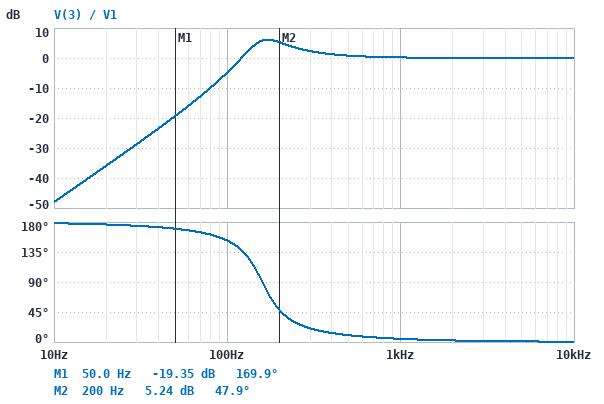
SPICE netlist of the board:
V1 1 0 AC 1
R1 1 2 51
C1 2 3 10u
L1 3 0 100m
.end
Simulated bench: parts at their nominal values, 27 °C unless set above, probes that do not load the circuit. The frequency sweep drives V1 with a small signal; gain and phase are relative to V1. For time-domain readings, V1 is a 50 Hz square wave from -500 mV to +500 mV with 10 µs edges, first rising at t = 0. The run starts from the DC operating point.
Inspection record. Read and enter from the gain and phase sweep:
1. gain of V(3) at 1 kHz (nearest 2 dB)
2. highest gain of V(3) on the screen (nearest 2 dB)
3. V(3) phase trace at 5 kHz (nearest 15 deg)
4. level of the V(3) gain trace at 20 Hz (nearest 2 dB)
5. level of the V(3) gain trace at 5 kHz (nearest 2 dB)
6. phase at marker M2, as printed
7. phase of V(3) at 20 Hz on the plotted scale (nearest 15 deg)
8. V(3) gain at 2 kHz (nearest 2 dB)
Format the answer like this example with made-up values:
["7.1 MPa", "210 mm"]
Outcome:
["0 dB", "6 dB", "0 deg", "-36 dB", "0 dB", "47.9 deg", "180 deg", "0 dB"]
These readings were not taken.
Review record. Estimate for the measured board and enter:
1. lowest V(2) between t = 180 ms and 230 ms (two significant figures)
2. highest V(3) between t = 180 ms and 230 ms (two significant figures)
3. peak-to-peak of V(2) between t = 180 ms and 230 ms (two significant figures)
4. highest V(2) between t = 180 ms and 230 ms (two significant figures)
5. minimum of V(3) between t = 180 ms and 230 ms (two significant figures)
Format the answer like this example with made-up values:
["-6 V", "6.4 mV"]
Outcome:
["-670 mV", "1.1 V", "1.3 V", "670 mV", "-1.1 V"]
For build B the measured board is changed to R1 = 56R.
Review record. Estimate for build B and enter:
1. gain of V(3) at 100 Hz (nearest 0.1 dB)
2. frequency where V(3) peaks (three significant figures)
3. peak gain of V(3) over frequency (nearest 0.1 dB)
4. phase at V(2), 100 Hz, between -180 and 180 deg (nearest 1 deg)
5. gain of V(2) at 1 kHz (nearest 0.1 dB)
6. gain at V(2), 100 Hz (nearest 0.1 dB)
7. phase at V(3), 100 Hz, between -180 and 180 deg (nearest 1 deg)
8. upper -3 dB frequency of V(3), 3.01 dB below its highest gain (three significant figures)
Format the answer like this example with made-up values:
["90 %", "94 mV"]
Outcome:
["-5.0 dB", "173 Hz", "5.4 dB", "-30 deg", "0 dB", "-1.3 dB", "150 deg", "288 Hz"]
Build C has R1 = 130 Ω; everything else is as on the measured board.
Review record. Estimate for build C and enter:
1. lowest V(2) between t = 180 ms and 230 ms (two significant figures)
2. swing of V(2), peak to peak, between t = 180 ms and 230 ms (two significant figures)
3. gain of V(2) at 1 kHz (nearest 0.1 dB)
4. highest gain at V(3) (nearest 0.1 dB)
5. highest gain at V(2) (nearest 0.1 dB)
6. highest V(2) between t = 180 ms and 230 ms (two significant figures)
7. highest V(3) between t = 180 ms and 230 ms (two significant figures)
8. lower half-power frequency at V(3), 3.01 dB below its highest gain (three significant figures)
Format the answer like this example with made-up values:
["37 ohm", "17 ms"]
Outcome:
["-540 mV", "1.1 V", "-0.2 dB", "0.1 dB", "0 dB", "540 mV", "990 mV", "149 Hz"]
